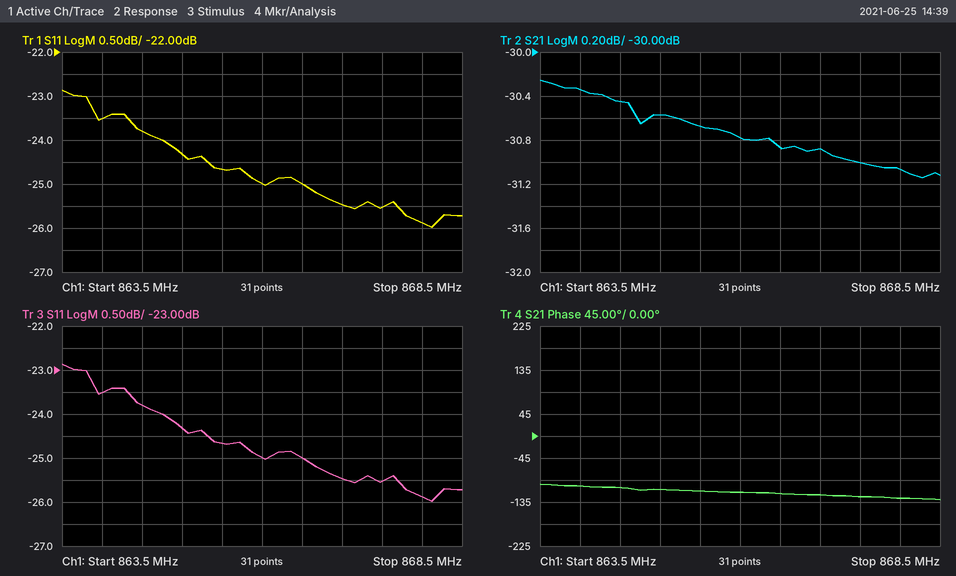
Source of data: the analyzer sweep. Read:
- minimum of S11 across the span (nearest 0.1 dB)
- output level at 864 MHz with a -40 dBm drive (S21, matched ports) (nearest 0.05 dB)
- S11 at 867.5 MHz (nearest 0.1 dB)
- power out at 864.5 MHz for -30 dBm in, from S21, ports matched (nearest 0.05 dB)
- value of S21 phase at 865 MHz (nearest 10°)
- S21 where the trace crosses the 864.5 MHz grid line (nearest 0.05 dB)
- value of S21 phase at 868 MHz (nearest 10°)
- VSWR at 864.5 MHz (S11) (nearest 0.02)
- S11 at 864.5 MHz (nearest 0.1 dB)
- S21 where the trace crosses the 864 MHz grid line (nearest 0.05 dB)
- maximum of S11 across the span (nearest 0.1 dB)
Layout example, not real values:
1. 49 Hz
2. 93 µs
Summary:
1. -26.0 dB
2. -70.35 dBm
3. -25.5 dB
4. -60.45 dBm
5. -110°
6. -30.45 dB
7. -130°
8. 1.14
9. -23.8 dB
10. -30.35 dB
11. -22.9 dB
